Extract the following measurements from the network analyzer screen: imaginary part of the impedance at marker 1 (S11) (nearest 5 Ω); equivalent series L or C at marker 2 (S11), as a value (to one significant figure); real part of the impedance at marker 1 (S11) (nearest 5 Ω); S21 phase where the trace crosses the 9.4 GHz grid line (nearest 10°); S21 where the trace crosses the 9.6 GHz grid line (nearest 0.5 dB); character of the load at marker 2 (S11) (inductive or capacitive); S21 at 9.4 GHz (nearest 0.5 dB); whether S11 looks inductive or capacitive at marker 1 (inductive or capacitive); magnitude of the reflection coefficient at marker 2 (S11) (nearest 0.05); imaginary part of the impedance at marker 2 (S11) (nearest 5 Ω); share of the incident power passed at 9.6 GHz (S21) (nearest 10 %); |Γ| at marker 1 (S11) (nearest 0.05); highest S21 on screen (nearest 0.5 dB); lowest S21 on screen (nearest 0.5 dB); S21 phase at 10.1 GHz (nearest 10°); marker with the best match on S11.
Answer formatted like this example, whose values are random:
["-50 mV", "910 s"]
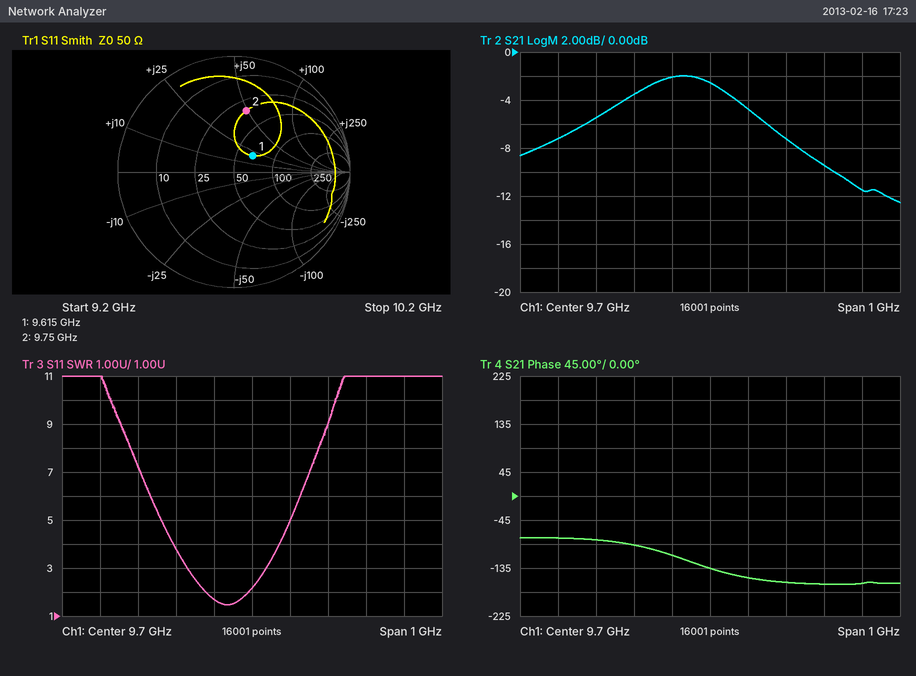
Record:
["+20 Ω", "800 pH", "65 Ω", "-80°", "-2.0 dB", "inductive", "-5.5 dB", "inductive", "0.55", "+50 Ω", "60 %", "0.20", "-2.0 dB", "-12.5 dB", "-160°", "marker 1"]
